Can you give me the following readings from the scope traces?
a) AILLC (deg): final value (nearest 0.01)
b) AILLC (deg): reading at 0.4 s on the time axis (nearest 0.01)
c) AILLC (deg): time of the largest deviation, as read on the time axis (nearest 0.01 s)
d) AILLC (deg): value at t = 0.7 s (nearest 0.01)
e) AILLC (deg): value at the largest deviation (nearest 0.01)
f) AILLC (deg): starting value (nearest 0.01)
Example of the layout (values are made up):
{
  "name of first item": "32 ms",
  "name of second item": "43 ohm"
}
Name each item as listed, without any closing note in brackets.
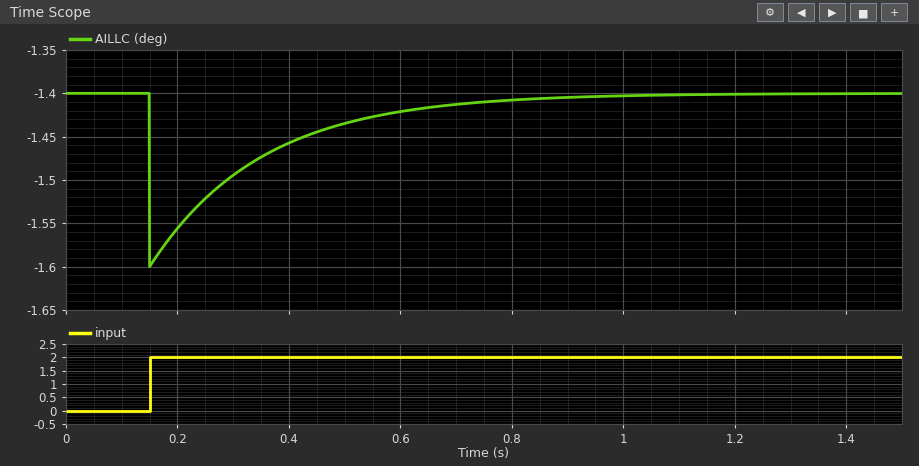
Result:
{
  "AILLC (deg): final value": "-1.40",
  "AILLC (deg): reading at 0.4 s on the time axis": "-1.46",
  "AILLC (deg): time of the largest deviation, as read on the time axis": "0.15 s",
  "AILLC (deg): value at t = 0.7 s": "-1.41",
  "AILLC (deg): value at the largest deviation": "-1.60",
  "AILLC (deg): starting value": "-1.40"
}
